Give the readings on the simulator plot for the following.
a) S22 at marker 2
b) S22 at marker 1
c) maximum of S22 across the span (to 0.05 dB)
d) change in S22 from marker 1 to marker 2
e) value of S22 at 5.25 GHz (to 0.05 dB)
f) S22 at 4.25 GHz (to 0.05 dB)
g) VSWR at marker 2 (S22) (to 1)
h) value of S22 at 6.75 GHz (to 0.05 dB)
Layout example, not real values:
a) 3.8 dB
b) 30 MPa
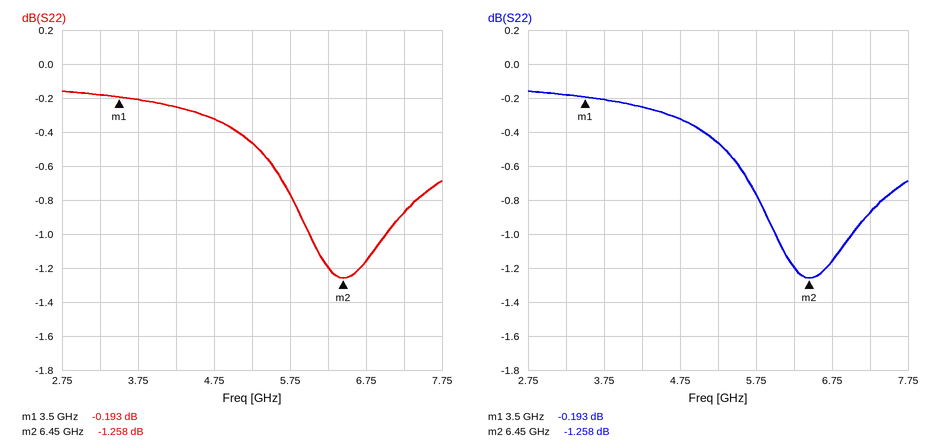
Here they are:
a) -1.258 dB
b) -0.193 dB
c) -0.15 dB
d) -1.065 dB
e) -0.45 dB
f) -0.25 dB
g) 14
h) -1.15 dB
